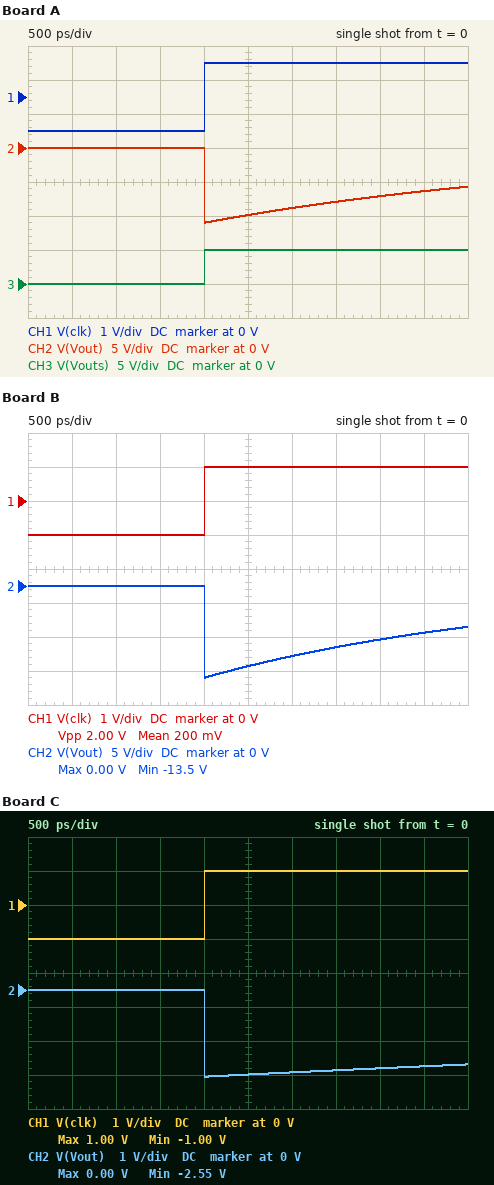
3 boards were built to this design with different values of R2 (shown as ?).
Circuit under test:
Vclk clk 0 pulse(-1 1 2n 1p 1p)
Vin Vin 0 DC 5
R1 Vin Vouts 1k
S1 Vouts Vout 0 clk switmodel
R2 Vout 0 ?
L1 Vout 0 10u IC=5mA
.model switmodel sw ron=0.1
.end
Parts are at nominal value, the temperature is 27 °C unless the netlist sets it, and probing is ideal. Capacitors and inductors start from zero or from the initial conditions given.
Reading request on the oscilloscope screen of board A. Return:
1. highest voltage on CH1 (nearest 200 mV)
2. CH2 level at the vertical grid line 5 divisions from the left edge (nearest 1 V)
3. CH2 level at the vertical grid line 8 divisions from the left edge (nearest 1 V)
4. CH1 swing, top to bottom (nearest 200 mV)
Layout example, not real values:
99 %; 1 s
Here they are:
1.0 V; -10 V; -7 V; 2.0 V
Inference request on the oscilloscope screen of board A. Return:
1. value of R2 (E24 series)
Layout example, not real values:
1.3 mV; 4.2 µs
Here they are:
2.2 kΩ
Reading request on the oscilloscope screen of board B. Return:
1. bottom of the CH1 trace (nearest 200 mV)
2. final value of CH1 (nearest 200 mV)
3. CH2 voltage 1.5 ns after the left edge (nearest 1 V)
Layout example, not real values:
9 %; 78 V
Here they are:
-1.0 V; 1.0 V; 0 V
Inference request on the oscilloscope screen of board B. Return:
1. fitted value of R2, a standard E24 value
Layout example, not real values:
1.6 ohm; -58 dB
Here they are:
2.7 kΩ
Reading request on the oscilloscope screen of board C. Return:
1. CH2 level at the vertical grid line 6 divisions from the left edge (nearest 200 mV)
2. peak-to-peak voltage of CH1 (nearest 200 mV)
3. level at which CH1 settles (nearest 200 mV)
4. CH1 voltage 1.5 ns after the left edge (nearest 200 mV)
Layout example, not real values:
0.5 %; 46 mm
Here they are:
-2.4 V; 2.0 V; 1.0 V; -1.0 V
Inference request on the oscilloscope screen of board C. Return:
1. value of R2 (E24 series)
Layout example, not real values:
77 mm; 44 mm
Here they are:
510 Ω
